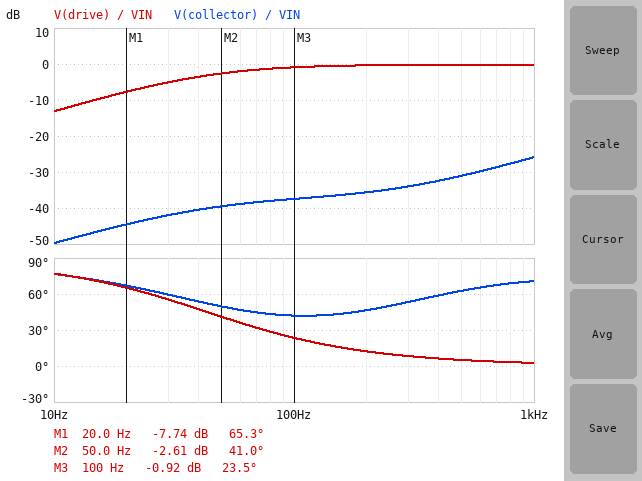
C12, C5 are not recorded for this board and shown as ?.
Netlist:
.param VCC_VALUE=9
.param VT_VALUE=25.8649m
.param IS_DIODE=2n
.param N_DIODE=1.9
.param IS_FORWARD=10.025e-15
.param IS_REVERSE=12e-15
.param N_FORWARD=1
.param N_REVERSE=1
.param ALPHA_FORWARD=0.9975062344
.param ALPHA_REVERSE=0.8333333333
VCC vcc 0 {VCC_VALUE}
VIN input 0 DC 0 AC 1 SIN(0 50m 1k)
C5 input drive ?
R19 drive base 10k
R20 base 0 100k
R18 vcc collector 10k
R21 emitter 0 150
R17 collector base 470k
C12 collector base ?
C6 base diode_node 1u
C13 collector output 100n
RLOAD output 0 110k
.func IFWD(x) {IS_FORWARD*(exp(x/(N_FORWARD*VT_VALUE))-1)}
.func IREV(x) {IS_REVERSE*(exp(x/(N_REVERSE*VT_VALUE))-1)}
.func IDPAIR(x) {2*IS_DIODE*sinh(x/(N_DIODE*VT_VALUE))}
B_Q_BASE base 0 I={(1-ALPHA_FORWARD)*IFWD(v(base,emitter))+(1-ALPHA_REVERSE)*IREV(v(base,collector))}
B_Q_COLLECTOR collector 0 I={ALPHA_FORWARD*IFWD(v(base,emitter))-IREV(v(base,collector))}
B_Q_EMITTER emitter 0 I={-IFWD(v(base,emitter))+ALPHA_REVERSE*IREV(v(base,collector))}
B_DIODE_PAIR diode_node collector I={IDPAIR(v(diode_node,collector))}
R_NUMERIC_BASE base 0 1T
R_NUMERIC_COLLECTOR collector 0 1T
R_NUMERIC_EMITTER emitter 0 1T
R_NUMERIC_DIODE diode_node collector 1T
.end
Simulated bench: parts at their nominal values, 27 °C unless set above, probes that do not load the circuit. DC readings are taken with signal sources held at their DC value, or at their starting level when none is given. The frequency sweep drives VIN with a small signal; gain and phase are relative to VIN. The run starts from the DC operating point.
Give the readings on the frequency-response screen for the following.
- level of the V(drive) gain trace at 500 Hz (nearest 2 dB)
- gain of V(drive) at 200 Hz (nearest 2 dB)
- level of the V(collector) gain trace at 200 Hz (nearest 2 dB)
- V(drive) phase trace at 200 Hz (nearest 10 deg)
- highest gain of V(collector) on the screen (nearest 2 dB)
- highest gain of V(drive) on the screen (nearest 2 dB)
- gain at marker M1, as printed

0 dB
0 dB
-36 dB
10 deg
-26 dB
0 dB
-7.74 dB
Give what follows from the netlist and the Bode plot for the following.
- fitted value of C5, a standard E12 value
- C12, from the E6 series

39 nF
1 nF
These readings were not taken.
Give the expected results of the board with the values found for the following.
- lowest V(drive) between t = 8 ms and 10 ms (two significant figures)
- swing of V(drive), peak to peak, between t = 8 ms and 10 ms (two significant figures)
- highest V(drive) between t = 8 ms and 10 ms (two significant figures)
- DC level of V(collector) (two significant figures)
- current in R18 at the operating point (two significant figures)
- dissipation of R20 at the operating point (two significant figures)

1.5 V
98 mV
1.6 V
8.8 V
16 µA
24 µW
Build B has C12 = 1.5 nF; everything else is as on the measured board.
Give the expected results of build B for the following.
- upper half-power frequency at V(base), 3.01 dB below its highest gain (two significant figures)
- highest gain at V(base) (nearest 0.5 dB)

9.5 kHz
-1.5 dB
